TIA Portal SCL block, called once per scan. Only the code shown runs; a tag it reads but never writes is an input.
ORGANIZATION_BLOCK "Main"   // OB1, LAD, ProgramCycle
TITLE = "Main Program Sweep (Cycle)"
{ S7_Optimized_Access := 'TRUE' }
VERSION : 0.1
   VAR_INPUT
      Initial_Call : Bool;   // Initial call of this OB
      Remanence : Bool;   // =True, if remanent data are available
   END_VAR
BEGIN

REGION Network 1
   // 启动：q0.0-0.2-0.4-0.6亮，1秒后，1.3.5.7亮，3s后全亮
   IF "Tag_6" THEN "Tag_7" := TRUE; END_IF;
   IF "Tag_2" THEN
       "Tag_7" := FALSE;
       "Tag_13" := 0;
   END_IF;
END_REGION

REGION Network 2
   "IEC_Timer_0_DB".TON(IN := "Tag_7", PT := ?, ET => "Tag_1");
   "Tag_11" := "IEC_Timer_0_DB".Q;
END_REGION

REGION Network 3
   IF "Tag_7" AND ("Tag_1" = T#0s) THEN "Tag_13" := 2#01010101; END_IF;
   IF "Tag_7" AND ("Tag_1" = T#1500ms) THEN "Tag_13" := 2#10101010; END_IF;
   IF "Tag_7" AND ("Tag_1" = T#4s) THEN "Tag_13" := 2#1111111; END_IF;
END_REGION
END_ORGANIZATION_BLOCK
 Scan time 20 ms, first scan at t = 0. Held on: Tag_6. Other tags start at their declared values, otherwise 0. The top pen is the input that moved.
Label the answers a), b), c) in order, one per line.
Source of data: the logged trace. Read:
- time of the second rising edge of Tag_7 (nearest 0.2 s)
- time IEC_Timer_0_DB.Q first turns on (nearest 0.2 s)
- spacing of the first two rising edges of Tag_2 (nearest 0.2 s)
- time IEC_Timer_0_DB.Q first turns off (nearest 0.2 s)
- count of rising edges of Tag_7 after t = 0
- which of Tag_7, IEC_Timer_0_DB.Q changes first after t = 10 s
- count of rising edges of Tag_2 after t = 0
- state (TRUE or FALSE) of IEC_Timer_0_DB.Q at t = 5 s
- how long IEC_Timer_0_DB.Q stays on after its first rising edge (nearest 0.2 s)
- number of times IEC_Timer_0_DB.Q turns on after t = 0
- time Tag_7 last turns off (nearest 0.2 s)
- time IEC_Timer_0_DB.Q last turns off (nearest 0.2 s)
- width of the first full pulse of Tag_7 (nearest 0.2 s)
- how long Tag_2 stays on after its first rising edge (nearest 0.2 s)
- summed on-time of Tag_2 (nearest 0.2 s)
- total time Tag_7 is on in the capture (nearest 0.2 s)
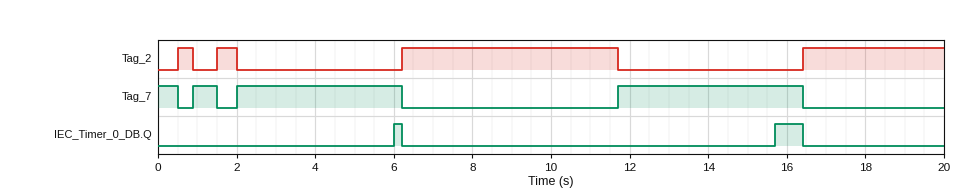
a) 2.0 s
b) 6.0 s
c) 1.0 s
d) 6.2 s
e) 3
f) Tag_7
g) 4
h) FALSE
i) 0.2 s
j) 2
k) 16.4 s
l) 16.4 s
m) 0.6 s
n) 0.4 s
o) 10.0 s
p) 10.0 s
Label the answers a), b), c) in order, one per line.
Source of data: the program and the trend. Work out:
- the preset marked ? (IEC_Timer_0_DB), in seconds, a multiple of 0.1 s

a) 4.0 s
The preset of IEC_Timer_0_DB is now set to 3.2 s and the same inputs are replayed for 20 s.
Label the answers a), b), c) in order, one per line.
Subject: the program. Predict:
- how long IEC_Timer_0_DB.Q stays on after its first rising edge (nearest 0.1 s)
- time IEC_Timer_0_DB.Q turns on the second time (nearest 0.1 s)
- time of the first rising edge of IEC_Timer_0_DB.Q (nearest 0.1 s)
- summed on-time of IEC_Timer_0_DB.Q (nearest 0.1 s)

a) 1.0 s
b) 14.9 s
c) 5.2 s
d) 2.5 s
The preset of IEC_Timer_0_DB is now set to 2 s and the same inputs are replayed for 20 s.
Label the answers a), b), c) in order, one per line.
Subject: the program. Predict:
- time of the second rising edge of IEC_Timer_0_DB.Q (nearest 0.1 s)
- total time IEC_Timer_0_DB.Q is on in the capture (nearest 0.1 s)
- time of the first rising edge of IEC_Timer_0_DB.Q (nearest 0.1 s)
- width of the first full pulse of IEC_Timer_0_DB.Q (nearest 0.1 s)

a) 13.7 s
b) 4.9 s
c) 4.0 s
d) 2.2 s
